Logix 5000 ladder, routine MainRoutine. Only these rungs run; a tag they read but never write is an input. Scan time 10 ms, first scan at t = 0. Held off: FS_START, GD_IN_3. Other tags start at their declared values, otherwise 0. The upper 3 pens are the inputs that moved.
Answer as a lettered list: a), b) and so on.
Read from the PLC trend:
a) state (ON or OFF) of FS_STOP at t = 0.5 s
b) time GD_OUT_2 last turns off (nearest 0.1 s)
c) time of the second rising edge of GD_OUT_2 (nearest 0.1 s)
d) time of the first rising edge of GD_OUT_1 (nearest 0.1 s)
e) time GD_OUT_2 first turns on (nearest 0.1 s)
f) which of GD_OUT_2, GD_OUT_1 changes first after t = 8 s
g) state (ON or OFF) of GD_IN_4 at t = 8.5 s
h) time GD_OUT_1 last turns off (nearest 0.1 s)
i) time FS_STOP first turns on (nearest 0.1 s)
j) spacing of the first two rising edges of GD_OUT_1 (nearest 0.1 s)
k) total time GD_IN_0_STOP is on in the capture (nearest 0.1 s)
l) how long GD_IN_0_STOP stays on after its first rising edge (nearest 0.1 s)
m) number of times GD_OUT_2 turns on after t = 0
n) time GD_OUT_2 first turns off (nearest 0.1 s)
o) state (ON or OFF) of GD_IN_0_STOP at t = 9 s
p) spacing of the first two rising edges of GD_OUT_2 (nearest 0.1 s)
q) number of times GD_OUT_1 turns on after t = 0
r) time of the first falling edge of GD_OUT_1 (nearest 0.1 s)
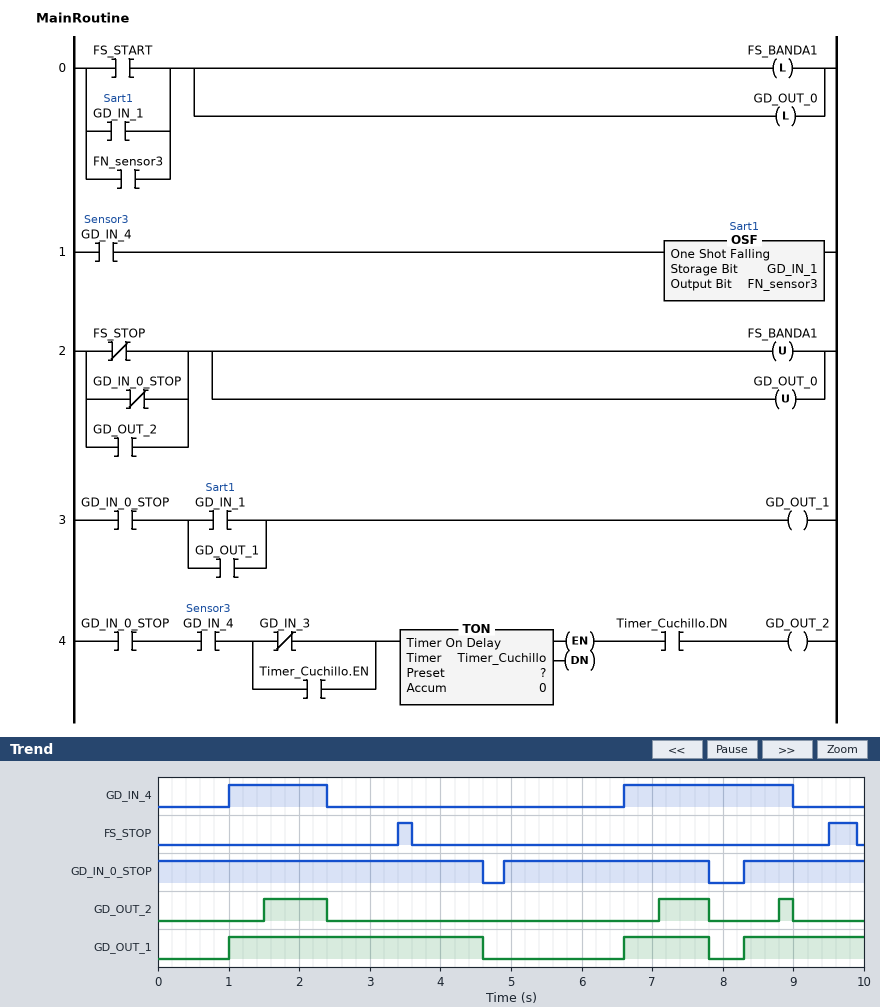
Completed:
a) OFF
b) 9.0 s
c) 7.1 s
d) 1.0 s
e) 1.5 s
f) GD_OUT_1
g) ON
h) 7.8 s
i) 3.4 s
j) 5.6 s
k) 9.2 s
l) 2.9 s
m) 3
n) 2.4 s
o) ON
p) 5.6 s
q) 3
r) 4.6 s
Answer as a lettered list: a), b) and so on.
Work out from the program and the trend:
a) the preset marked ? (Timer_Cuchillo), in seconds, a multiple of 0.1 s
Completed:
a) 0.5 s
